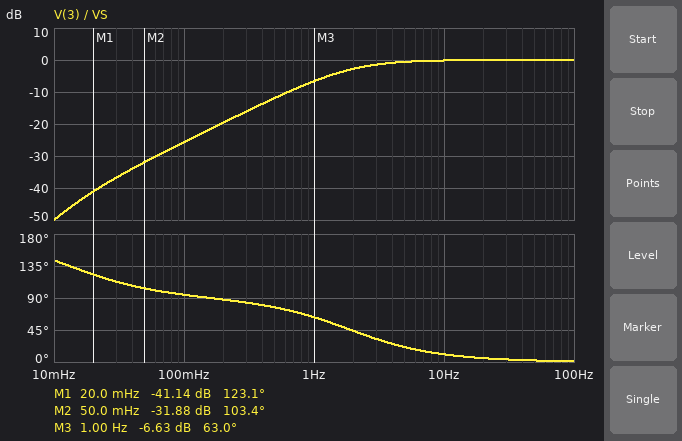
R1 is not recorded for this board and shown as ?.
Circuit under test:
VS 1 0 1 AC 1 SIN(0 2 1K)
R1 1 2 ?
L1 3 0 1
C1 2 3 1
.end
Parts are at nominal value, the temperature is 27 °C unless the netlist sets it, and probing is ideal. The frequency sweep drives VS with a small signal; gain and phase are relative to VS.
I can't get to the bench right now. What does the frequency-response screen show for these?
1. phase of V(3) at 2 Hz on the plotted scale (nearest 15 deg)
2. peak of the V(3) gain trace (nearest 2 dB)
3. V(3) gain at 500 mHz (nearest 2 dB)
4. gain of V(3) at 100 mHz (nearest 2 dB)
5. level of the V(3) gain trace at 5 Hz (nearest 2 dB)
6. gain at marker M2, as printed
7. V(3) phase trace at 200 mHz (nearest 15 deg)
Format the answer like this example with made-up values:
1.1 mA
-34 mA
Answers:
45 deg
0 dB
-12 dB
-26 dB
0 dB
-31.88 dB
90 deg
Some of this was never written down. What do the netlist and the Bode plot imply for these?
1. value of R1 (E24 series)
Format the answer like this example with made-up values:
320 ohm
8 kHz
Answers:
12 Ω
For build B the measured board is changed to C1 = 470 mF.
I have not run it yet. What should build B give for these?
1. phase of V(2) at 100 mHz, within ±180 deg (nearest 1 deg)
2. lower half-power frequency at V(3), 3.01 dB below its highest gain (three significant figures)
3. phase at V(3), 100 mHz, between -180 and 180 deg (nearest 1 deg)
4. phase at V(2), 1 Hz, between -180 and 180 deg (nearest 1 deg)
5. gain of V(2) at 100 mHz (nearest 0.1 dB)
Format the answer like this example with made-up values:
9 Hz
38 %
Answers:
-77 deg
1.88 Hz
103 deg
64 deg
-13.0 dB
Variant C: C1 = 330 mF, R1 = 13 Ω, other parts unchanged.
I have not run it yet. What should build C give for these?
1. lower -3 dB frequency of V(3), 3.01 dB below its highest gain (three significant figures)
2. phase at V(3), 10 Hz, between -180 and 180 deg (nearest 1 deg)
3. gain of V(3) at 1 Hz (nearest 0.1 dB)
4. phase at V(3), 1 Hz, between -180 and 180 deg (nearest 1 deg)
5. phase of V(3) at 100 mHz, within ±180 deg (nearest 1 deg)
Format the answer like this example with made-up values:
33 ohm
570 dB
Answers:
2.03 Hz
12 deg
-7.1 dB
66 deg
108 deg
